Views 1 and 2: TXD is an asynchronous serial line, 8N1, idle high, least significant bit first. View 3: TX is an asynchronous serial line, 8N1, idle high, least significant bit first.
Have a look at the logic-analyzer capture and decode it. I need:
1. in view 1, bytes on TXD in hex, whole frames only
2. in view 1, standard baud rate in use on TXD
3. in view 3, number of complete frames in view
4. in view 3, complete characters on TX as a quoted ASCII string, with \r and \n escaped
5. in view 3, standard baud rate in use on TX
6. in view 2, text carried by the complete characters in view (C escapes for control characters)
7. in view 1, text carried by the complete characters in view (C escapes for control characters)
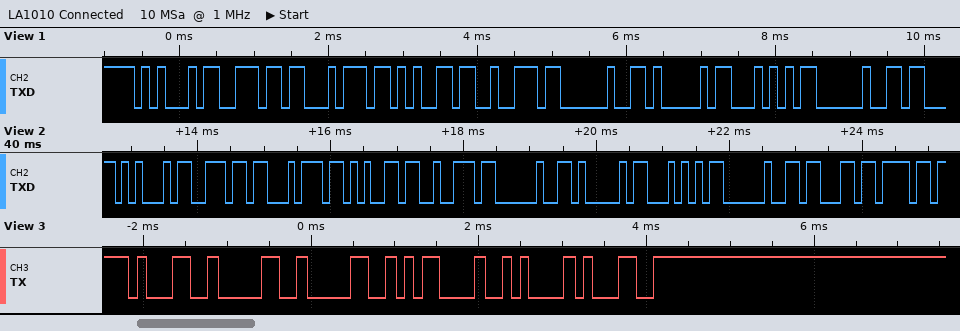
45 6E 74 65 72 20 41 54 20
9600 baud
6
"100\r\n1"
9600 baud
"Enter AT co"
"Enter AT "
